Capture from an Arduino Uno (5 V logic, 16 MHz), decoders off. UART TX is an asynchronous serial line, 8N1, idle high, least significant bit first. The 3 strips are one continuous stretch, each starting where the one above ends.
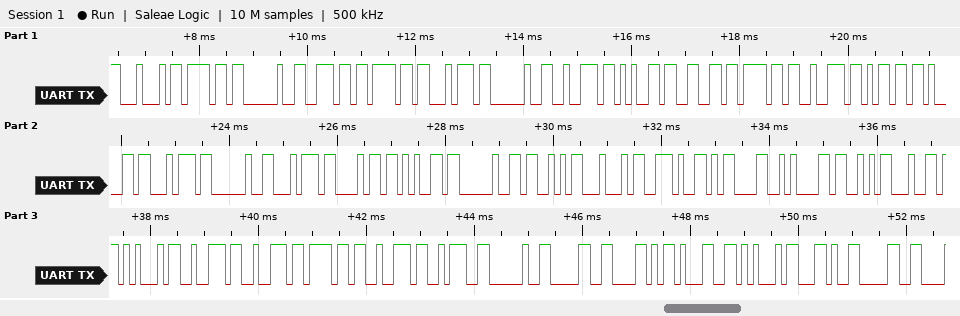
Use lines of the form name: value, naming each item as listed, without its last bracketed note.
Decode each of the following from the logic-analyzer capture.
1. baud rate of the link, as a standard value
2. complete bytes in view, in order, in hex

baud rate of the link, as a standard value: 9600 baud
complete bytes in view, in order, in hex: 0x44 0x6F 0x20 0x6E 0x6F 0x74 0x20 0x72 0x65 0x66 0x6F 0x72 0x6D 0x61 0x74 0x20 0x74 0x68 0x65 0x20 0x53 0x44 0x2E 0x0D 0x0A 0x53 0x64 0x45 0x72 0x72 0x6F 0x72 0x3A 0x20 0x30 0x58 0x31 0x45 0x2C 0x30
